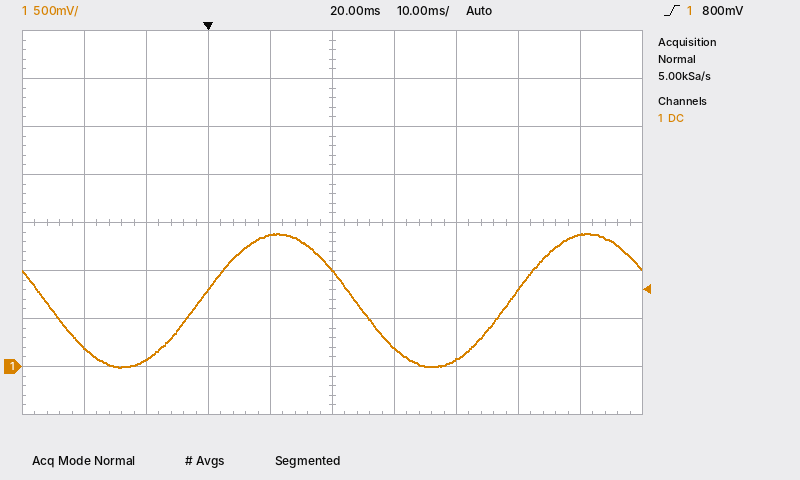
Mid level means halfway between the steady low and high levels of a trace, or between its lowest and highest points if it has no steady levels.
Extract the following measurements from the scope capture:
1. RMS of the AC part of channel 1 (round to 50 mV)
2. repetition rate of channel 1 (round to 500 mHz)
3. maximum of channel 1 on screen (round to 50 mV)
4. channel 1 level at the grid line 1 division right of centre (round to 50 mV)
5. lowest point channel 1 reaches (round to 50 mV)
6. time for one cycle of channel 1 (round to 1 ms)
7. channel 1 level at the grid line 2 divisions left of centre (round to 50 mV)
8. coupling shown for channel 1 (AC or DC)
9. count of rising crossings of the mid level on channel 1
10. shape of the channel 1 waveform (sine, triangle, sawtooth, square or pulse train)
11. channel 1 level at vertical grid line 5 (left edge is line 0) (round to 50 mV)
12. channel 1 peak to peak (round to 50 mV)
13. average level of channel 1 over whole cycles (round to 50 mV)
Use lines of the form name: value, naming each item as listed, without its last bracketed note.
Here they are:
RMS of the AC part of channel 1: 500 mV
repetition rate of channel 1: 20.0 Hz
maximum of channel 1 on screen: 1.40 V
channel 1 level at the grid line 1 division right of centre: 200 mV
lowest point channel 1 reaches: 0 mV
time for one cycle of channel 1: 50 ms
channel 1 level at the grid line 2 divisions left of centre: 800 mV
coupling shown for channel 1: DC
count of rising crossings of the mid level on channel 1: 2
shape of the channel 1 waveform: sine
channel 1 level at vertical grid line 5 (left edge is line 0): 1.00 V
channel 1 peak to peak: 1.40 V
average level of channel 1 over whole cycles: 700 mV
